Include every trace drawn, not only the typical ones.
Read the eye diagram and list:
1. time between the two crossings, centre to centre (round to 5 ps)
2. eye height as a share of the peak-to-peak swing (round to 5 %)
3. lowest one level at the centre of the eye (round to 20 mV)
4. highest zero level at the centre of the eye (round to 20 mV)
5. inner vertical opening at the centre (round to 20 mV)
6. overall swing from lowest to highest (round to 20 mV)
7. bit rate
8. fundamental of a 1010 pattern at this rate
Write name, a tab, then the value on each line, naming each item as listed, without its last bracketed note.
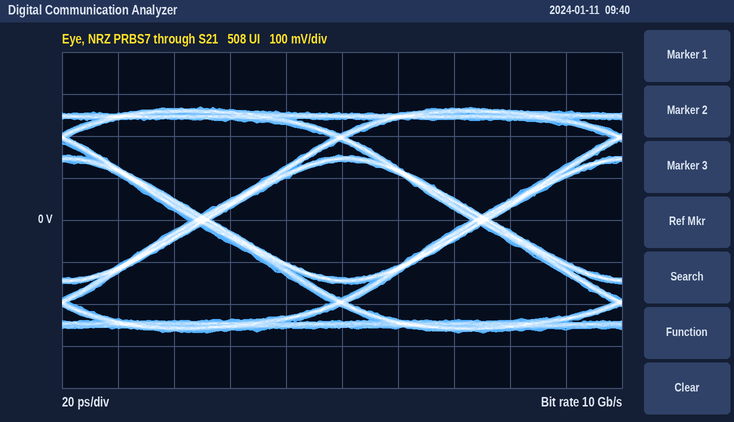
time between the two crossings, centre to centre	100 ps
eye height as a share of the peak-to-peak swing	50 %
lowest one level at the centre of the eye	140 mV
highest zero level at the centre of the eye	-140 mV
inner vertical opening at the centre	280 mV
overall swing from lowest to highest	540 mV
bit rate	10 Gb/s
fundamental of a 1010 pattern at this rate	5 GHz
